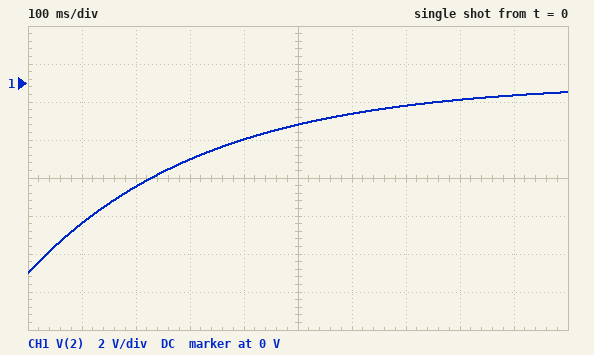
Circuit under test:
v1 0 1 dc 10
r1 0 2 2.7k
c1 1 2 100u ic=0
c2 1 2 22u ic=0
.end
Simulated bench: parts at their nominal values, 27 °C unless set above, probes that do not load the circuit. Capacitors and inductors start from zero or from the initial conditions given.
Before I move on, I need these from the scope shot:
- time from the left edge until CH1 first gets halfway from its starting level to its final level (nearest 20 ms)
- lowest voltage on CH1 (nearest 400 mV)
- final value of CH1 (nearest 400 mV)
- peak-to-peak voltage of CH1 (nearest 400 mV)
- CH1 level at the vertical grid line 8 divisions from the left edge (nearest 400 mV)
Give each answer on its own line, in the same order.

220 ms
-10.0 V
-400 mV
9.6 V
-800 mV
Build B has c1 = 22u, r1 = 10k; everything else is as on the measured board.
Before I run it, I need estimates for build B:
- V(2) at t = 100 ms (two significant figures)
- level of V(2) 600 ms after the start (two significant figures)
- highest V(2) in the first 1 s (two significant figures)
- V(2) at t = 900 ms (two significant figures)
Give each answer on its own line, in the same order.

-8.0 V
-2.6 V
-1.0 V
-1.3 V
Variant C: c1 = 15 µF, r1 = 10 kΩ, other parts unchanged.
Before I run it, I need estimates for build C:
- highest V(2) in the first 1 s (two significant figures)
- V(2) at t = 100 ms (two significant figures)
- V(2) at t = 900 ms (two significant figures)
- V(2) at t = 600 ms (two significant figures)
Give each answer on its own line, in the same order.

-670 mV
-7.6 V
-880 mV
-2.0 V
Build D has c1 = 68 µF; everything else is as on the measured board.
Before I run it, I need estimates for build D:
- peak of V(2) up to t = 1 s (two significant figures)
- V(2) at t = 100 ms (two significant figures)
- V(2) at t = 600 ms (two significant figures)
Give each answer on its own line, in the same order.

-160 mV
-6.6 V
-850 mV
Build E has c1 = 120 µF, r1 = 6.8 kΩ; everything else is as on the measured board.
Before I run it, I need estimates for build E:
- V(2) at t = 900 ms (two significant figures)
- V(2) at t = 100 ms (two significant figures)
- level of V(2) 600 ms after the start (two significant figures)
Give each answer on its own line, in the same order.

-3.9 V
-9.0 V
-5.4 V
